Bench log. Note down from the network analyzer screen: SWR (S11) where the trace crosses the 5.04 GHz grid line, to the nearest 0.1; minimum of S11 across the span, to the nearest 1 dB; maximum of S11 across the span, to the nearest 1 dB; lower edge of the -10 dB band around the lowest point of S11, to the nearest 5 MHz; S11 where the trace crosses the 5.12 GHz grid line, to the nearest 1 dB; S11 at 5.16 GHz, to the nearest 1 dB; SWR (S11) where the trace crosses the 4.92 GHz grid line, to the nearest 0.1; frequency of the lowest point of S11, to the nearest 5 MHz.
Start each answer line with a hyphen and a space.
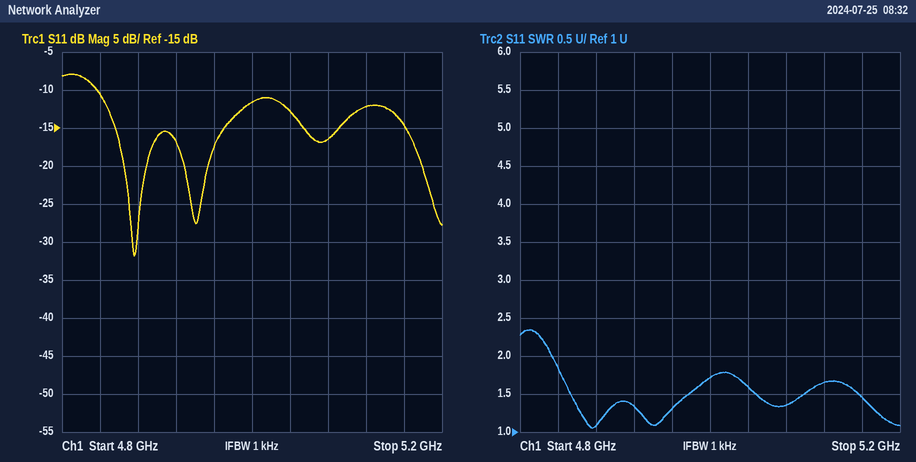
- 1.6
- -32 dB
- -8 dB
- 4.835 GHz
- -12 dB
- -15 dB
- 1.3
- 4.875 GHz
